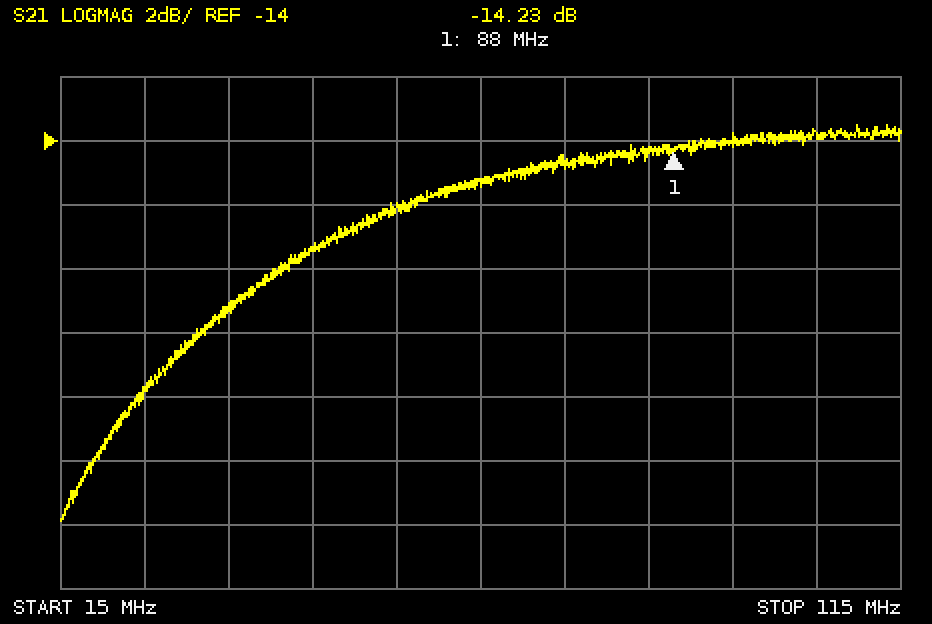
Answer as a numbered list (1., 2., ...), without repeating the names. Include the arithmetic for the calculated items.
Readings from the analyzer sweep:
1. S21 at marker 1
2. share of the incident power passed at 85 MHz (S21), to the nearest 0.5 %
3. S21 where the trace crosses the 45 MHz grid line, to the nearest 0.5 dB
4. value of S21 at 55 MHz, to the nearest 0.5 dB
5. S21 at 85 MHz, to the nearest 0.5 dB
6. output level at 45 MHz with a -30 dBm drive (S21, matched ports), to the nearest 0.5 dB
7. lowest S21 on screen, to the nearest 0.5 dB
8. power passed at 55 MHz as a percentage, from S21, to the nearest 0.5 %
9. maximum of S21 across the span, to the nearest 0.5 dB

1. -14.23 dB
2. 10^(-14.5/10) ≈ 3.5 %
3. -17.5 dB
4. -16.0 dB
5. -14.5 dB
6. -30 dBm + (-17.5 dB) = -47.5 dBm
7. -26.0 dB
8. 10^(-16/10) ≈ 2.5 %
9. -13.5 dB
